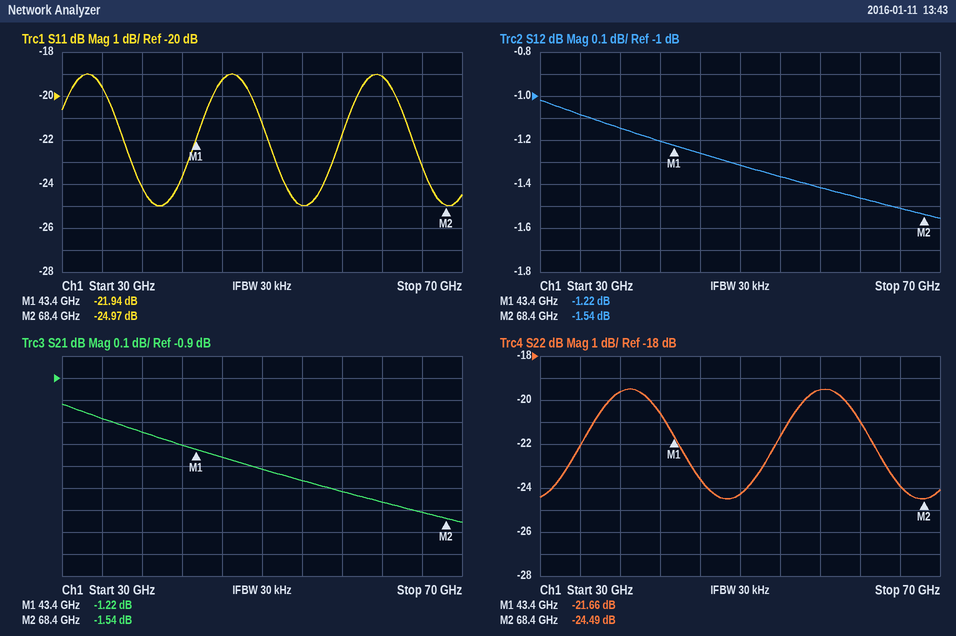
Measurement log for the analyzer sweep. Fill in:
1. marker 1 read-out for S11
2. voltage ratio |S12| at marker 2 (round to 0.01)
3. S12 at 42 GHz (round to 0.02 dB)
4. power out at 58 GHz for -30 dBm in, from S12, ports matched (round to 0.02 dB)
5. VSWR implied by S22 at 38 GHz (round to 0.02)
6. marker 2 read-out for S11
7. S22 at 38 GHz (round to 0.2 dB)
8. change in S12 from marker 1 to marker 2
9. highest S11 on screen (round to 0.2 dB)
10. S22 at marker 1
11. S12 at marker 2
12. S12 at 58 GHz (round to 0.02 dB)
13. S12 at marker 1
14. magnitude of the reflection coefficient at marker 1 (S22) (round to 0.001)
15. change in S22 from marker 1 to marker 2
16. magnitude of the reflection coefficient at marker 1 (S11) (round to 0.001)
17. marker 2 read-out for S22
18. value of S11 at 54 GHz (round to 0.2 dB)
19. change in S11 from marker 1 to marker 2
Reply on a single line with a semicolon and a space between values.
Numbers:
-21.94 dB; 0.84; -1.20 dB; -31.42 dBm; 1.24; -24.97 dB; -19.6 dB; -0.32 dB; -19.0 dB; -21.66 dB; -1.54 dB; -1.42 dB; -1.22 dB; 0.083; -2.83 dB; 0.080; -24.49 dB; -25.0 dB; -3.03 dB
